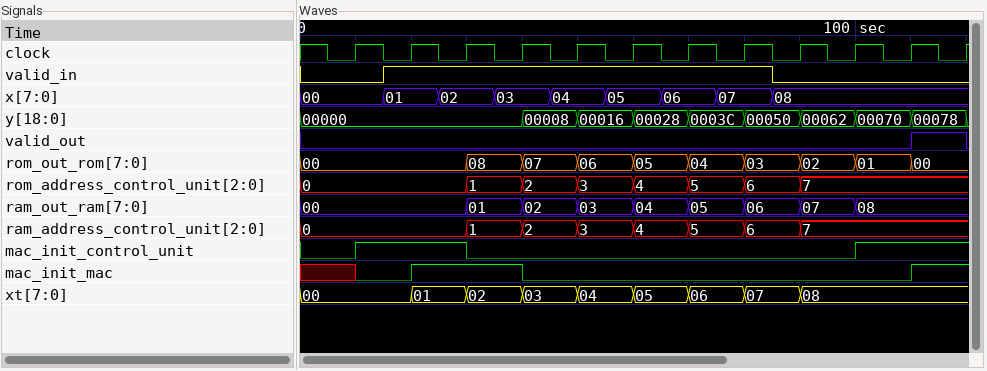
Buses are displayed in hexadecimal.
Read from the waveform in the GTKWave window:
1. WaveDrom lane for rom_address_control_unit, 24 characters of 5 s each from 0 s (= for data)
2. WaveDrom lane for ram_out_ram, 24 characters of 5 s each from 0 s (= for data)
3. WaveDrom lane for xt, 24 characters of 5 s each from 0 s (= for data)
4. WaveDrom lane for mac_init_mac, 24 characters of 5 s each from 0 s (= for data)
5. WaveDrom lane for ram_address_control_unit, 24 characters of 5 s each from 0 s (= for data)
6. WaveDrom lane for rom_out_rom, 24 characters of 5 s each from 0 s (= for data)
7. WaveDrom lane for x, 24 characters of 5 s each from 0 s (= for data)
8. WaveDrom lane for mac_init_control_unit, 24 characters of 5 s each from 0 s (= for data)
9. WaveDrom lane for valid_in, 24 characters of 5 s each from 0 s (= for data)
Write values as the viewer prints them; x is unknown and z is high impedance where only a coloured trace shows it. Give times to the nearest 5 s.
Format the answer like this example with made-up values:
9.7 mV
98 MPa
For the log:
{name: 'rom_address_control_unit', wave: '=.....=.=.=.=.=.=.=.....', data: '0 1 2 3 4 5 6 7'}
{name: 'ram_out_ram', wave: '=.....=.=.=.=.=.=.=.=...', data: '00 01 02 03 04 05 06 07 08'}
{name: 'xt', wave: '=...=.=.=.=.=.=.=.=.....', data: '00 01 02 03 04 05 06 07 08'}
{name: 'mac_init_mac', wave: 'x.0.1...0.............1.'}
{name: 'ram_address_control_unit', wave: '=.....=.=.=.=.=.=.=.....', data: '0 1 2 3 4 5 6 7'}
{name: 'rom_out_rom', wave: '=.....=.=.=.=.=.=.=.=.=.', data: '00 08 07 06 05 04 03 02 01 00'}
{name: 'x', wave: '=..=.=.=.=.=.=.=.=......', data: '00 01 02 03 04 05 06 07 08'}
{name: 'mac_init_control_unit', wave: '0.1...0.............1...'}
{name: 'valid_in', wave: '0..1.............0......'}
